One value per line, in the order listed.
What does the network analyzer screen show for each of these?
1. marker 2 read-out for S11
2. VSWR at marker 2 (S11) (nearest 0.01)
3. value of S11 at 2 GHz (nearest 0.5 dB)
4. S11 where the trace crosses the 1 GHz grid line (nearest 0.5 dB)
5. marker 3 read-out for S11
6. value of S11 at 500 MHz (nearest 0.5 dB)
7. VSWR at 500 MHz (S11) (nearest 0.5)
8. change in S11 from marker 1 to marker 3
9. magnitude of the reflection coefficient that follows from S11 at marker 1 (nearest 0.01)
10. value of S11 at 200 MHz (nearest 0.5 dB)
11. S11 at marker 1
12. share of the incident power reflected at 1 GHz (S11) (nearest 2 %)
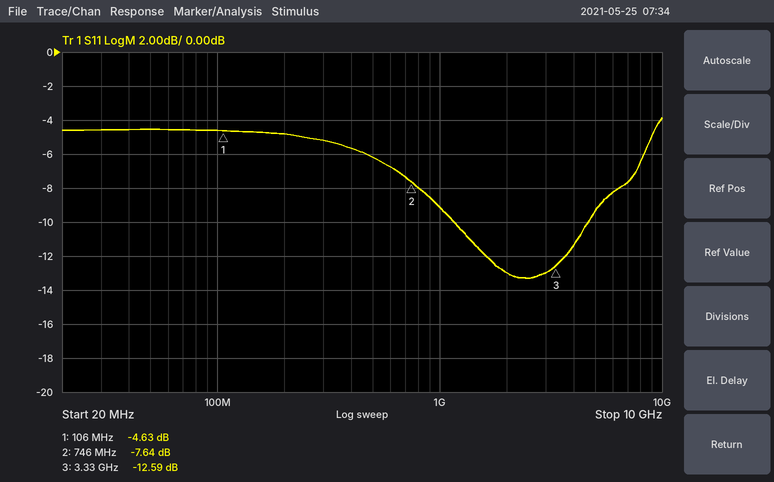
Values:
-7.64 dB
2.42
-13.0 dB
-9.0 dB
-12.59 dB
-6.0 dB
3.0
-7.96 dB
0.59
-5.0 dB
-4.63 dB
12 %
